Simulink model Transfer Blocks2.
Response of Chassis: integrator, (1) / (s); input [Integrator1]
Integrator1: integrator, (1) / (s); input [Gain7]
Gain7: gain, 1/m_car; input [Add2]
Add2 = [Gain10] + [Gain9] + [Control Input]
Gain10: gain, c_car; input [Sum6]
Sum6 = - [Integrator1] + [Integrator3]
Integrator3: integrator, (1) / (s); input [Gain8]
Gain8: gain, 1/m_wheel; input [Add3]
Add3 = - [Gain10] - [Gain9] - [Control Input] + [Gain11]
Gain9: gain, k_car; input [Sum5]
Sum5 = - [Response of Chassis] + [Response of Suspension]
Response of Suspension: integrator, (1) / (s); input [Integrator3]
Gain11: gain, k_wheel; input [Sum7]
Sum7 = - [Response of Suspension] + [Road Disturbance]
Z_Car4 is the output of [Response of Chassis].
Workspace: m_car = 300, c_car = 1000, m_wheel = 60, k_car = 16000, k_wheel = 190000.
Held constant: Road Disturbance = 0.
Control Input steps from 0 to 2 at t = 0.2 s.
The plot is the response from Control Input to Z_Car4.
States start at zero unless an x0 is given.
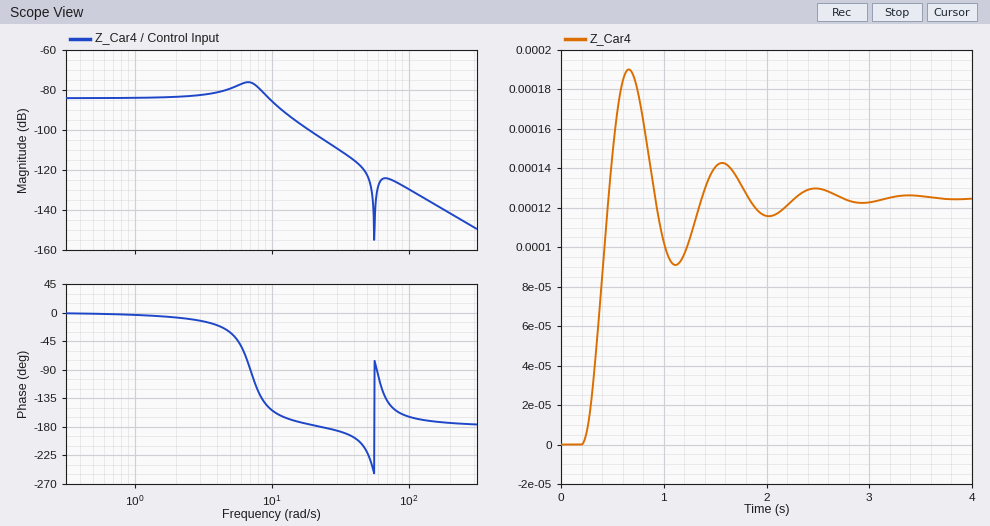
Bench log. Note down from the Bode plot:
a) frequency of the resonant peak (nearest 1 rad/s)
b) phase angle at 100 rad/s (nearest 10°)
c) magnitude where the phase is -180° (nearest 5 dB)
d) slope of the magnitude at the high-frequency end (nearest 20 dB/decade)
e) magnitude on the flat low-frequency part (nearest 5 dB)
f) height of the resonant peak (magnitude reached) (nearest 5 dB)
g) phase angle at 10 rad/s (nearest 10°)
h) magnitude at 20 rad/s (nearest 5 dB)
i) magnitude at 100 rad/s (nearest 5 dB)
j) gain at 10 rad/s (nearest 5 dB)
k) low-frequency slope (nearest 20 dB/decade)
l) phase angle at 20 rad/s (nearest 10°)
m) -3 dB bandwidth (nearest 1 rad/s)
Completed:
7 rad/s
-160°
-105 dB
-40 dB/decade
-85 dB
-75 dB
-150°
-100 dB
-130 dB
-85 dB
0 dB/decade
-180°
11 rad/s
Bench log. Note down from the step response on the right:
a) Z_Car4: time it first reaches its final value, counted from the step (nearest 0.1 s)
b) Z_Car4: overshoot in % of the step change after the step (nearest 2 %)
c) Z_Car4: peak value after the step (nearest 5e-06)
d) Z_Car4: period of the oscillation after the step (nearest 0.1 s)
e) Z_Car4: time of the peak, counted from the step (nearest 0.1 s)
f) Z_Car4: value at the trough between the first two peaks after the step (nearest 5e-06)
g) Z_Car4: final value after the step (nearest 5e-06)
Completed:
0.3 s
52 %
0.000190
0.9 s
0.5 s
0.000090
0.000125
